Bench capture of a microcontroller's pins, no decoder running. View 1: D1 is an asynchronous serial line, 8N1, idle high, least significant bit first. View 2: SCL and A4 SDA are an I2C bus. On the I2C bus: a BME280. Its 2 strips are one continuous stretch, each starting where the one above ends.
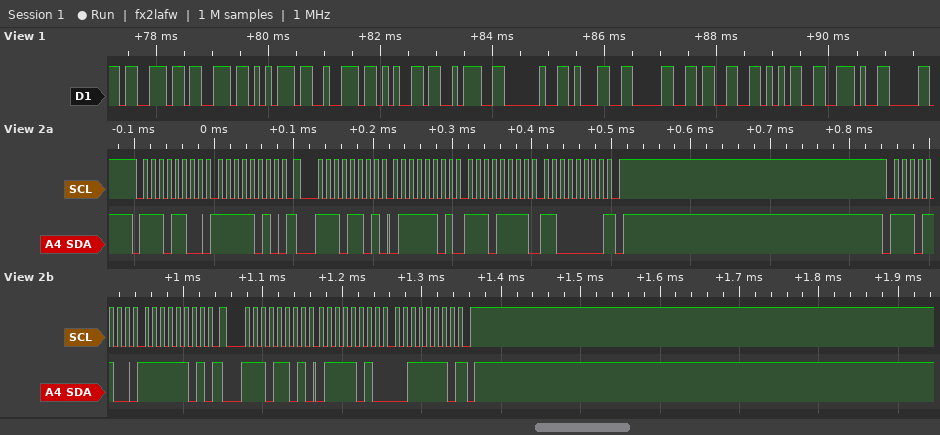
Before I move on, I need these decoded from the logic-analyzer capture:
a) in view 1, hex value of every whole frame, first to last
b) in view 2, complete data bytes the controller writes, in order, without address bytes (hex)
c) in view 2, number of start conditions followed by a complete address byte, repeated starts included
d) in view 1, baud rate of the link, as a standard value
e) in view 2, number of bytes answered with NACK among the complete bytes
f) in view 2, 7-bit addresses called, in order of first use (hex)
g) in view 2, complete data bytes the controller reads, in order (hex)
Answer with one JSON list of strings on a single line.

["73 73 75 72 65 3A 20 31 30 33 35 2E", "FA FD", "4", "9600 baud", "2", "0x76", "7D EF C0 7A 3E"]
